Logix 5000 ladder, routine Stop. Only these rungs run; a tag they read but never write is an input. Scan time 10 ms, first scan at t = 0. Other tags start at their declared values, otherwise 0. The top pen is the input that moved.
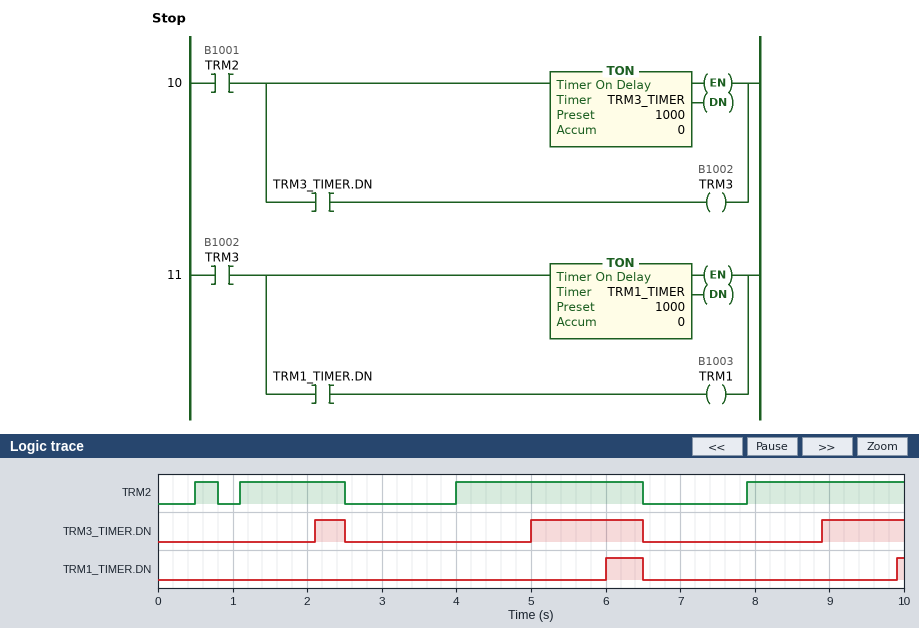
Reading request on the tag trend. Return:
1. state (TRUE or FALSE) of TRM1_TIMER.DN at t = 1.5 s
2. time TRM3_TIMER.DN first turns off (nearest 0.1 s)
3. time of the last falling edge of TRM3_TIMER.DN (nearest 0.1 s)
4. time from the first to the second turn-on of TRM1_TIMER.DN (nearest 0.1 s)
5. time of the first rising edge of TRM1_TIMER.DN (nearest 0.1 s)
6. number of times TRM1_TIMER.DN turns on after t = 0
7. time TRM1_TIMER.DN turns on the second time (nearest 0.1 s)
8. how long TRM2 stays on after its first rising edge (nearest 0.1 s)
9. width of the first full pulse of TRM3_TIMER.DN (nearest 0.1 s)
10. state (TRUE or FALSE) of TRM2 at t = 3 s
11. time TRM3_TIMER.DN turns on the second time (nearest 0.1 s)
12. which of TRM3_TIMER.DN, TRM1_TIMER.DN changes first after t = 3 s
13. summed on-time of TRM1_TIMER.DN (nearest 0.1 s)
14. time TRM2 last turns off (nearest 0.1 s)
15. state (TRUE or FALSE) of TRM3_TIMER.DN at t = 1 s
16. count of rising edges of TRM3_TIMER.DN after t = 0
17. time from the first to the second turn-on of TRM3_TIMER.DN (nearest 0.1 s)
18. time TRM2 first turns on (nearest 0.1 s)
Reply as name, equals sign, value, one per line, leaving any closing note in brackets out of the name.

state (TRUE or FALSE) of TRM1_TIMER.DN at t = 1.5 s = FALSE
time TRM3_TIMER.DN first turns off = 2.5 s
time of the last falling edge of TRM3_TIMER.DN = 6.5 s
time from the first to the second turn-on of TRM1_TIMER.DN = 3.9 s
time of the first rising edge of TRM1_TIMER.DN = 6.0 s
number of times TRM1_TIMER.DN turns on after t = 0 = 2
time TRM1_TIMER.DN turns on the second time = 9.9 s
how long TRM2 stays on after its first rising edge = 0.3 s
width of the first full pulse of TRM3_TIMER.DN = 0.4 s
state (TRUE or FALSE) of TRM2 at t = 3 s = FALSE
time TRM3_TIMER.DN turns on the second time = 5.0 s
which of TRM3_TIMER.DN, TRM1_TIMER.DN changes first after t = 3 s = TRM3_TIMER.DN
summed on-time of TRM1_TIMER.DN = 0.6 s
time TRM2 last turns off = 6.5 s
state (TRUE or FALSE) of TRM3_TIMER.DN at t = 1 s = FALSE
count of rising edges of TRM3_TIMER.DN after t = 0 = 3
time from the first to the second turn-on of TRM3_TIMER.DN = 2.9 s
time TRM2 first turns on = 0.5 s
